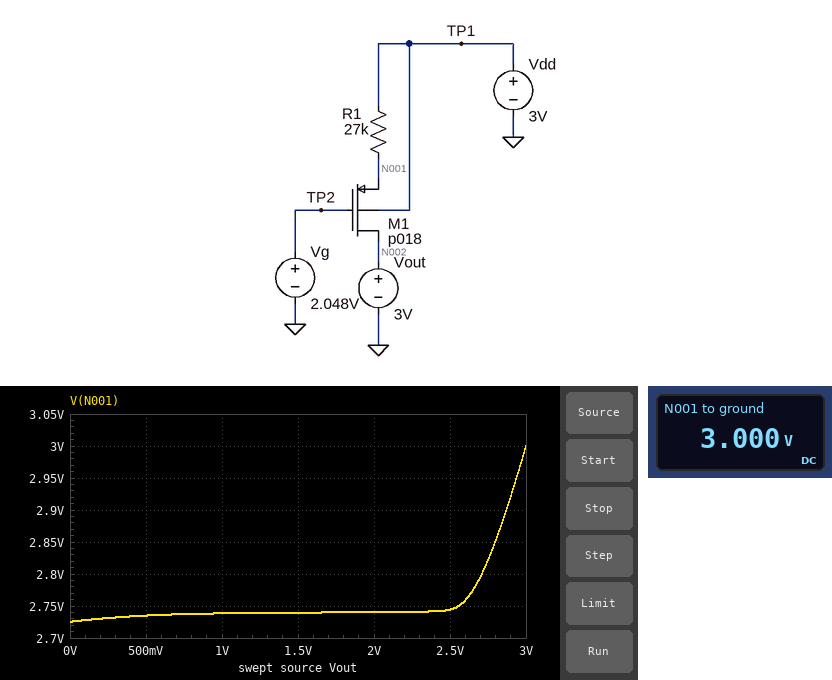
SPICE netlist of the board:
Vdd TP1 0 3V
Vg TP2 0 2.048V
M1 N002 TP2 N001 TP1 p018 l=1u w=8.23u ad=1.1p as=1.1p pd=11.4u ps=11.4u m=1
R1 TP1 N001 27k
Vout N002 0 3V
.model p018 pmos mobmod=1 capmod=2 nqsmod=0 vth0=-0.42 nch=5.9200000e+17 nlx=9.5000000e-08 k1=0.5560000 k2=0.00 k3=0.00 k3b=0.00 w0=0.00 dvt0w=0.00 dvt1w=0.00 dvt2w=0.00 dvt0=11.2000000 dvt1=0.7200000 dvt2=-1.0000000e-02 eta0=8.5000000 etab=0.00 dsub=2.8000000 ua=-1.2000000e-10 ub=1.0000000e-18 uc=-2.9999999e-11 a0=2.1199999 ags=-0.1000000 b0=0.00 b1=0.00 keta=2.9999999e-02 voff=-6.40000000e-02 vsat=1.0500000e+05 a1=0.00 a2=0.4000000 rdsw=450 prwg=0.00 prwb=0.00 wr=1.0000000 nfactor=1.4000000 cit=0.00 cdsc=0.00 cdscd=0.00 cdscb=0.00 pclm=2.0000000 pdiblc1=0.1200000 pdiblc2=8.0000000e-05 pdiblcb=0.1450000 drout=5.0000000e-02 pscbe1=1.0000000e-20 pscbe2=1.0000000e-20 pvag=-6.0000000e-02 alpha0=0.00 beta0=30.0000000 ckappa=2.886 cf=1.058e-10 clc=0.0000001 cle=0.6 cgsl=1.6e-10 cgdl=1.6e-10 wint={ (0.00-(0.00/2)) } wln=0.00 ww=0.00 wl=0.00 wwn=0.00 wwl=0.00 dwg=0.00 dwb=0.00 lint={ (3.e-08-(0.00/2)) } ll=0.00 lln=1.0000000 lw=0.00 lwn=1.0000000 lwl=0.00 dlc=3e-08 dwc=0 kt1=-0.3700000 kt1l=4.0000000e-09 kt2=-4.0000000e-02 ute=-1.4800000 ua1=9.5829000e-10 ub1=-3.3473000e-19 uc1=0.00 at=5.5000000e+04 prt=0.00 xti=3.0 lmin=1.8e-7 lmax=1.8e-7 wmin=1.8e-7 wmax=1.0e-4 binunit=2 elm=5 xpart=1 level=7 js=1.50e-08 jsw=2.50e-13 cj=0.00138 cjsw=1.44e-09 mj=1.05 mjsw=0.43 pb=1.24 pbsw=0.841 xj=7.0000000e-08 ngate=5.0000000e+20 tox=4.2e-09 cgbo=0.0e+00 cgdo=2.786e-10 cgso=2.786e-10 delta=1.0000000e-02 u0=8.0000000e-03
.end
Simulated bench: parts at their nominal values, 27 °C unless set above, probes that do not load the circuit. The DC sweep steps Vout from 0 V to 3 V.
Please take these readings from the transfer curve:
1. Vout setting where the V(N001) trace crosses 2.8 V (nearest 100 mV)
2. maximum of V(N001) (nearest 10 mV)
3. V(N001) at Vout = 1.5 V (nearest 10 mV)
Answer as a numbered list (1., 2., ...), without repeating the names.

1. 2.7 V
2. 3.00 V
3. 2.74 V
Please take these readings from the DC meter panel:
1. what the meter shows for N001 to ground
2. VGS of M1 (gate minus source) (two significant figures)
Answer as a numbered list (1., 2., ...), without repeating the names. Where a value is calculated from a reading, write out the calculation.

1. 3.000 V
2. 2.048 V - 3 V = -950 mV
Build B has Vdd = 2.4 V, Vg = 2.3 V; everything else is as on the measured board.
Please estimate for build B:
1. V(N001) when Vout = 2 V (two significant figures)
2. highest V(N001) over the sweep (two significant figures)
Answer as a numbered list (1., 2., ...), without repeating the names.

1. 2.4 V
2. 2.8 V
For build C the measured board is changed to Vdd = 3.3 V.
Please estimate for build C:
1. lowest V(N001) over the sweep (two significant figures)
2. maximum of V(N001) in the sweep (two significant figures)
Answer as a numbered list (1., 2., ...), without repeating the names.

1. 2.8 V
2. 3.1 V
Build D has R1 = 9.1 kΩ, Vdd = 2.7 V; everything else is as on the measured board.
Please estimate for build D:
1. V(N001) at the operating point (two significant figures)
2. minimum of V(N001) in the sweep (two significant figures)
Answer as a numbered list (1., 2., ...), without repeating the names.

1. 2.9 V
2. 2.6 V
